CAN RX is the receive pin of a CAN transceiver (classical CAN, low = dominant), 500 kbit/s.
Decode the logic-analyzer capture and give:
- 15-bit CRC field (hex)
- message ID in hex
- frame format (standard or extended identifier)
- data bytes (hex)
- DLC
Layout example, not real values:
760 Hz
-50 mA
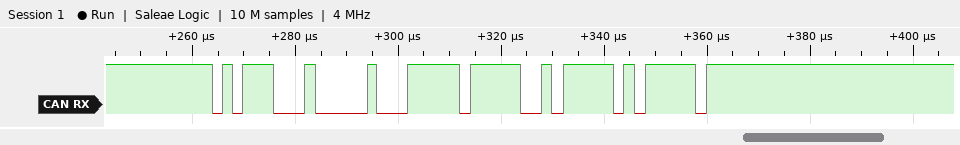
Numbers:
0x57EF
0x5C4
standard
FF
1
